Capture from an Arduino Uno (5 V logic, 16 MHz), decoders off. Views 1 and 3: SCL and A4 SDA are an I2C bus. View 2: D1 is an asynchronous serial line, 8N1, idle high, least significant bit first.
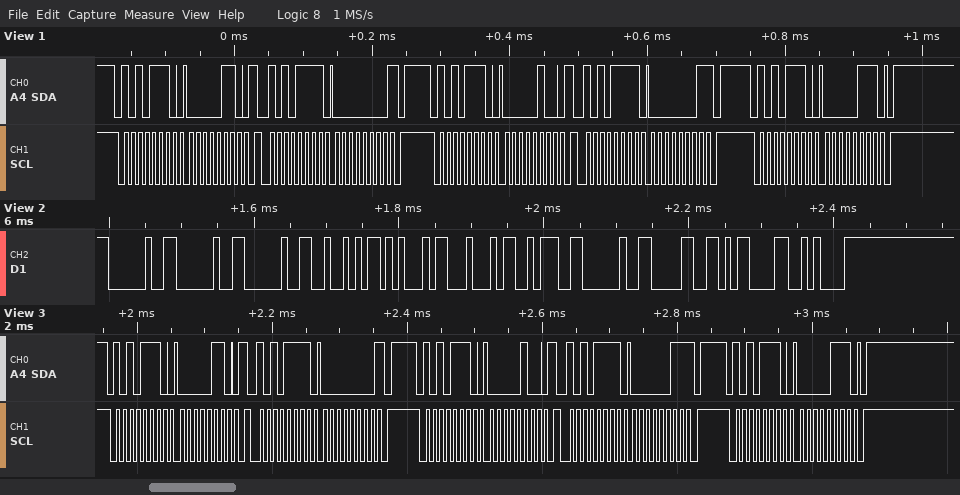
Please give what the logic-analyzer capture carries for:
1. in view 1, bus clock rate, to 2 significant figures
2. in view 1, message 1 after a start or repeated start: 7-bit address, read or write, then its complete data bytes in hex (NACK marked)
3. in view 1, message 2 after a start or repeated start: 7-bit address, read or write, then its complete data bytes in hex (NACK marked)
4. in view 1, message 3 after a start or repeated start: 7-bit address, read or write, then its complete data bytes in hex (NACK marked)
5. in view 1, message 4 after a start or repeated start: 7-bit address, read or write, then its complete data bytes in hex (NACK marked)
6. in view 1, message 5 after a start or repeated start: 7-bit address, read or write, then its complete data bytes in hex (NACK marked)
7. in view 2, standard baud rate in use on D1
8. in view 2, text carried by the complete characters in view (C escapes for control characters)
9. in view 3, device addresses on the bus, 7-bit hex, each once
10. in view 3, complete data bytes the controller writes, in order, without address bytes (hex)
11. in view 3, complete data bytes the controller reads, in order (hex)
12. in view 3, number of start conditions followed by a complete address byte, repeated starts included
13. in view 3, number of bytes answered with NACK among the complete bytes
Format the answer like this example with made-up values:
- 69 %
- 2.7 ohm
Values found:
- 100 kHz
- 0x57 write: 06
- 0x57 read: 00 NACK
- 0x57 write: 04
- 0x57 read: 01 NACK
- 0x57 write: 07
- 115200 baud
- "   RED: 0\r\n"
- 0x57
- 06 04 07
- 00 03
- 5
- 2
